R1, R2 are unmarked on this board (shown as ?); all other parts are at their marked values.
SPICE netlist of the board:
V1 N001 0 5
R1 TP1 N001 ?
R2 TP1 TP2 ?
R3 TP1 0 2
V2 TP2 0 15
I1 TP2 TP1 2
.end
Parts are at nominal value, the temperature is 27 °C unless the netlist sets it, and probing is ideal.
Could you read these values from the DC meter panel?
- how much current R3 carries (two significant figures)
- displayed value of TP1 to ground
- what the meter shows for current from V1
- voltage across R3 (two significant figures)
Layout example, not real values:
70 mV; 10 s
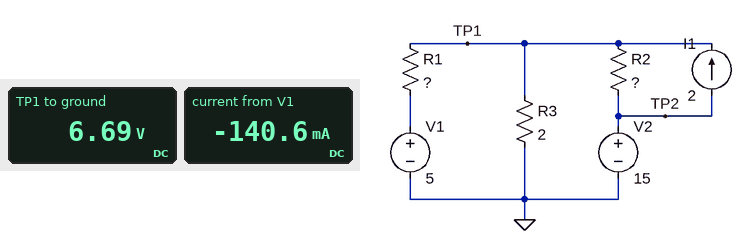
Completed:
3.3 A; 6.69 V; -140.6 mA; 6.7 V
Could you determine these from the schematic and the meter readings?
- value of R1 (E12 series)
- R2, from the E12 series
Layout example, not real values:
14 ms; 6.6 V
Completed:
12 Ω; 5.6 Ω
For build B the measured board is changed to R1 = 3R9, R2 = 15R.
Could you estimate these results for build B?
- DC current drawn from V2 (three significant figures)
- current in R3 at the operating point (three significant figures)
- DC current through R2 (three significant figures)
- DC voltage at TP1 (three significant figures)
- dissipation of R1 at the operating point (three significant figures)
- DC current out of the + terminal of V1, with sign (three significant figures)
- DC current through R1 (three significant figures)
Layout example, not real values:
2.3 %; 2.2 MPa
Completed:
2.65 A; 2.60 A; 653 mA; 5.20 V; 10.5 mW; -51.9 mA; 51.9 mA
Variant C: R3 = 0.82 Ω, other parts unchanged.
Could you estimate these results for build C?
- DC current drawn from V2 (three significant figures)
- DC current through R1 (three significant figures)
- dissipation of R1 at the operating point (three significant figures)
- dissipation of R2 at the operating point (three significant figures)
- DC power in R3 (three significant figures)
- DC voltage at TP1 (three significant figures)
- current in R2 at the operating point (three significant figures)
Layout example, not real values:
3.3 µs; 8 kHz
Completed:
4.06 A; 130 mA; 203 mW; 23.9 W; 14.4 W; 3.44 V; 2.06 A
